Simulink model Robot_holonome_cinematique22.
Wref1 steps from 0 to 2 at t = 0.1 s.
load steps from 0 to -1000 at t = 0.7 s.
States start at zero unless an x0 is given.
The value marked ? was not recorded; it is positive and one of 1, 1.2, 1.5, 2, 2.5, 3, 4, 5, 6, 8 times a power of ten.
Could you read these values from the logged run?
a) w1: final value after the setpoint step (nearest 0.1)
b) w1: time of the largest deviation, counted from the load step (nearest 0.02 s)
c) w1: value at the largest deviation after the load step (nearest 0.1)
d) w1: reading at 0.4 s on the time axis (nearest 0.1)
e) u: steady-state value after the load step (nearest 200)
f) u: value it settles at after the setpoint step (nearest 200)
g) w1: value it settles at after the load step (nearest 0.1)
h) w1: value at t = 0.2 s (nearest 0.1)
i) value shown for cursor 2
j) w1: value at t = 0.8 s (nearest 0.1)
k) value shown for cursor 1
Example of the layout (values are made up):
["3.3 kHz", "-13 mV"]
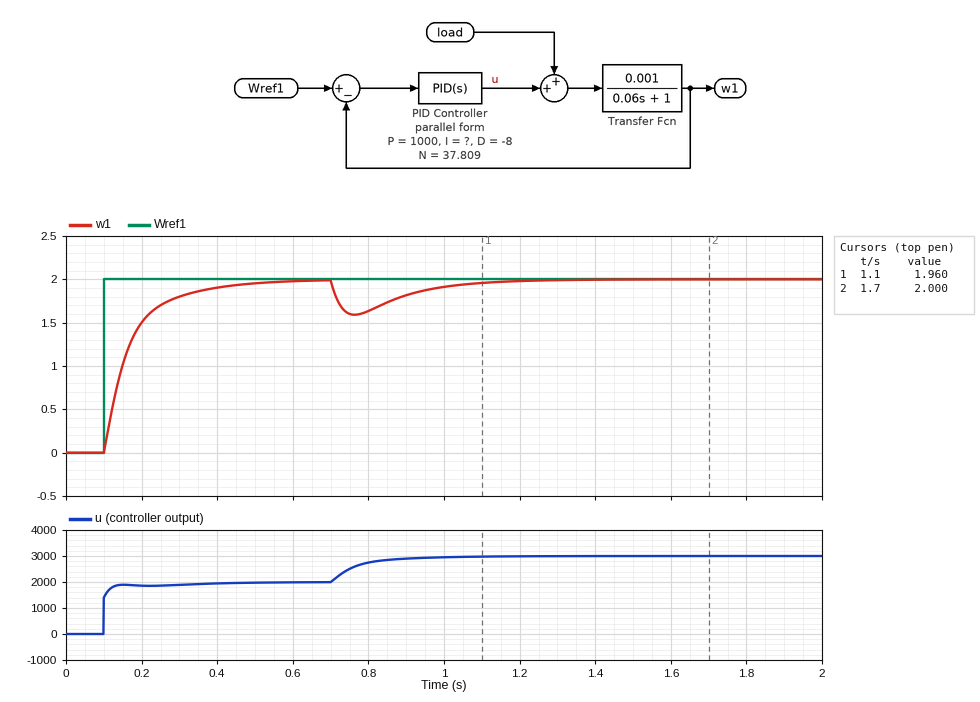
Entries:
["2.0", "0.06 s", "1.6", "1.9", "3000", "2000", "2.0", "1.5", "2.000", "1.6", "1.960"]
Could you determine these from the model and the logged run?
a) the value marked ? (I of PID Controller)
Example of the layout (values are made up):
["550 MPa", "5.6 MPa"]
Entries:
["12000"]
